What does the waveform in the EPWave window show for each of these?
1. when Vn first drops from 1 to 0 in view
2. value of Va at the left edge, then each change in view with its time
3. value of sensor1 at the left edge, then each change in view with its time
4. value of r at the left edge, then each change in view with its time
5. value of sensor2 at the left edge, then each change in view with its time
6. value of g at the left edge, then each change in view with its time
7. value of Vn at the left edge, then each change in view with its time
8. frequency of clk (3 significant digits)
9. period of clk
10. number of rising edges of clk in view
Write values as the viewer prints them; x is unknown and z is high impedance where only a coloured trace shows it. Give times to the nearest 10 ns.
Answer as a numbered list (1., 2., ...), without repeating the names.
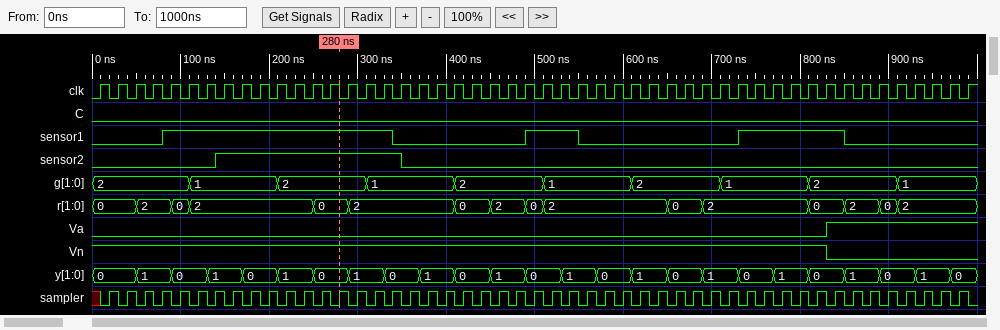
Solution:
1. 830 ns
2. 0, 1 at 830 ns
3. 0, 1 at 80 ns, 0 at 340 ns, 1 at 490 ns, 0 at 550 ns, 1 at 730 ns, 0 at 850 ns
4. 0, 2 at 50 ns, 0 at 90 ns, 2 at 110 ns, 0 at 250 ns, 2 at 290 ns, 0 at 410 ns, 2 at 450 ns, 0 at 490 ns, 2 at 510 ns, 0 at 650 ns, 2 at 690 ns, 0 at 810 ns, 2 at 850 ns, 0 at 890 ns, 2 at 910 ns
5. 0, 1 at 140 ns, 0 at 350 ns
6. 2, 1 at 110 ns, 2 at 210 ns, 1 at 310 ns, 2 at 410 ns, 1 at 510 ns, 2 at 610 ns, 1 at 710 ns, 2 at 810 ns, 1 at 910 ns
7. 1, 0 at 830 ns
8. 50.0 MHz
9. 20 ns
10. 50
